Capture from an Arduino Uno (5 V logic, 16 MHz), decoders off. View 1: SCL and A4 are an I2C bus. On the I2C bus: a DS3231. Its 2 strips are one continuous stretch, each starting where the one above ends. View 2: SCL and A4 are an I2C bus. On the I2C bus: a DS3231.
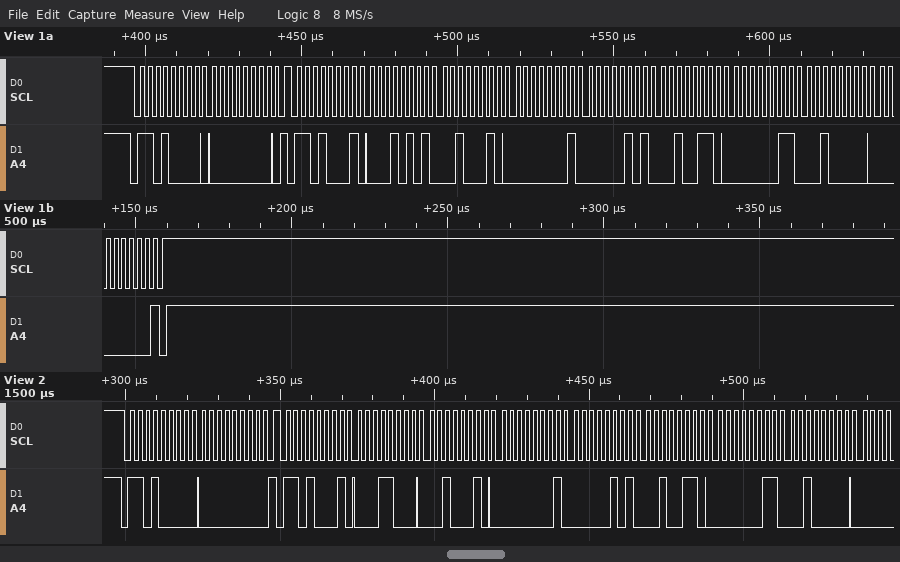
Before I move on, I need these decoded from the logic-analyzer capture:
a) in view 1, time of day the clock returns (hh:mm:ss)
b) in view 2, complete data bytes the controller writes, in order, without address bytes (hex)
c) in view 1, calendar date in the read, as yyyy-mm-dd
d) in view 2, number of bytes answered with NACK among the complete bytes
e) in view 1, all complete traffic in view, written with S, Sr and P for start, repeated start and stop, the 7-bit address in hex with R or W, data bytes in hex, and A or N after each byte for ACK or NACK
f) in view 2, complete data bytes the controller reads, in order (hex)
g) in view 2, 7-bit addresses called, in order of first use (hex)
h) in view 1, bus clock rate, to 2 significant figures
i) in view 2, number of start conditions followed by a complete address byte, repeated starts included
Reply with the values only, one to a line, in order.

01:22:15
00
2020-03-26
0
S 68W A 00 A Sr 68R A 15 A 22 A 01 A 05 A 26 A 03 A 20 A 00 N P
18 22 01 05 26 03 20
0x68
400 kHz
2
